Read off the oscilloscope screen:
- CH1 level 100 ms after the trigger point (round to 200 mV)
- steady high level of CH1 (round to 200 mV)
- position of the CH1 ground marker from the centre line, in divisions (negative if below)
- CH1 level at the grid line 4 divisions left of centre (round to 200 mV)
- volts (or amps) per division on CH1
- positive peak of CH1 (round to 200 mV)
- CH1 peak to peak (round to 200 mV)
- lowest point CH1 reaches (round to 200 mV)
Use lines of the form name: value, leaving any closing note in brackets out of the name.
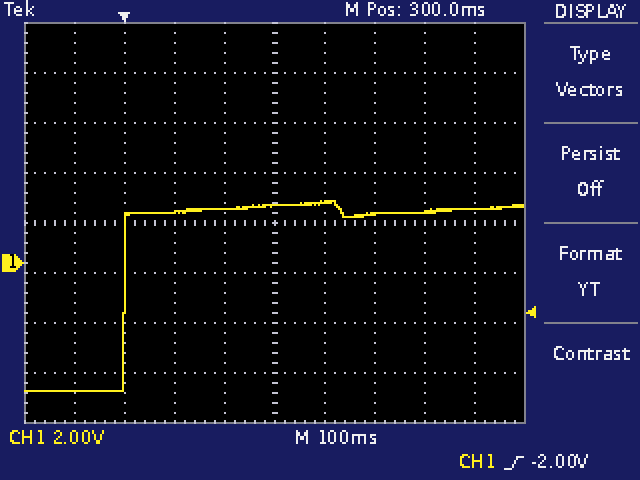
CH1 level 100 ms after the trigger point: 2.0 V
steady high level of CH1: 2.2 V
position of the CH1 ground marker from the centre line, in divisions: -0.8 div
CH1 level at the grid line 4 divisions left of centre: -5.2 V
volts (or amps) per division on CH1: 2 V
positive peak of CH1: 2.4 V
CH1 peak to peak: 7.6 V
lowest point CH1 reaches: -5.2 V
